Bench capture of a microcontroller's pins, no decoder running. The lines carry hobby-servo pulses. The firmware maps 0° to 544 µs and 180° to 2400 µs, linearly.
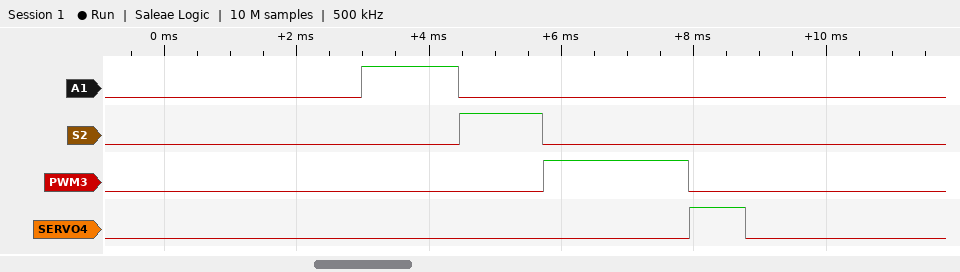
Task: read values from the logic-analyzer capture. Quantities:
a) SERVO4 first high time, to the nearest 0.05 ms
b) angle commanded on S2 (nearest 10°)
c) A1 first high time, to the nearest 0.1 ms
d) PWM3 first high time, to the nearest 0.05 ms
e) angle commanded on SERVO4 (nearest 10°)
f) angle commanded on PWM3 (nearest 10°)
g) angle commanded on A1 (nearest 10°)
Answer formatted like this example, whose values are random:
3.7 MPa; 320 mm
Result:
0.85 ms; 70°; 1.5 ms; 2.20 ms; 30°; 160°; 90°
